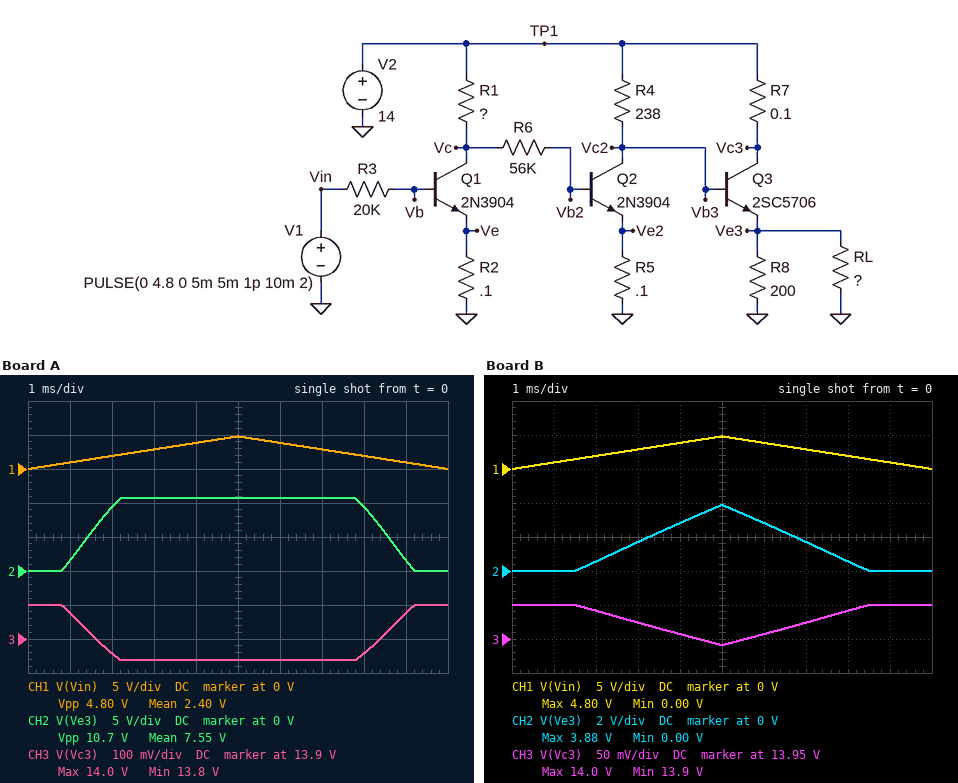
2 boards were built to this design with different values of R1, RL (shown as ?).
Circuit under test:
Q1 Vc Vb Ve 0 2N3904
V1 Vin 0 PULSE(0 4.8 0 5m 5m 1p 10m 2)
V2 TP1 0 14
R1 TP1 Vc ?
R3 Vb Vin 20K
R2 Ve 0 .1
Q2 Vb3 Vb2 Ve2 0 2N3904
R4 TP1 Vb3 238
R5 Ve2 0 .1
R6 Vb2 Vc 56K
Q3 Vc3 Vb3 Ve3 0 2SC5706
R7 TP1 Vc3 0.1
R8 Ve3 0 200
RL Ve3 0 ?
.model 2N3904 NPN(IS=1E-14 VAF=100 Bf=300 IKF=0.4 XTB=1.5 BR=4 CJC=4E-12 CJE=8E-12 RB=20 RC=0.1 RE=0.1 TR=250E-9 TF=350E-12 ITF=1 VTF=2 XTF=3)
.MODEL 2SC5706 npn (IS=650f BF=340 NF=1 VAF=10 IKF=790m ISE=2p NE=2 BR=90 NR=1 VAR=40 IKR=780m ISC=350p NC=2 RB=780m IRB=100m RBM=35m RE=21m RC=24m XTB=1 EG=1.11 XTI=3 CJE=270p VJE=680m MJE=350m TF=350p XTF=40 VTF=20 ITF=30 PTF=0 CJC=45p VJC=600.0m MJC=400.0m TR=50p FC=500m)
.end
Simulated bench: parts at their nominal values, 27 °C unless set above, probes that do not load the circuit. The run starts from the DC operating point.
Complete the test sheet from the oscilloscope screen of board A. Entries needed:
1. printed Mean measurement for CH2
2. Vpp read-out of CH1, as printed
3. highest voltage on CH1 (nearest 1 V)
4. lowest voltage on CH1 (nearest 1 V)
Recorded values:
7.55 V
4.80 V
5 V
0 V
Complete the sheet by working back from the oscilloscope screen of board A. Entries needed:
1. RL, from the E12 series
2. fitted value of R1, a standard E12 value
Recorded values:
6.8 Ω
680 Ω
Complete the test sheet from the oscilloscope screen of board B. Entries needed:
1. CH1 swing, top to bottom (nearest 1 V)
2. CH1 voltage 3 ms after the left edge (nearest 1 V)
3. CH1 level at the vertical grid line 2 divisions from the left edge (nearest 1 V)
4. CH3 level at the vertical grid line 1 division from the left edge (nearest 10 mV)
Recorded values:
5 V
3 V
2 V
14.00 V
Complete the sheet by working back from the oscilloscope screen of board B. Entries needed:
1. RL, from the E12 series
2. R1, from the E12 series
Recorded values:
6.8 Ω
100 Ω
